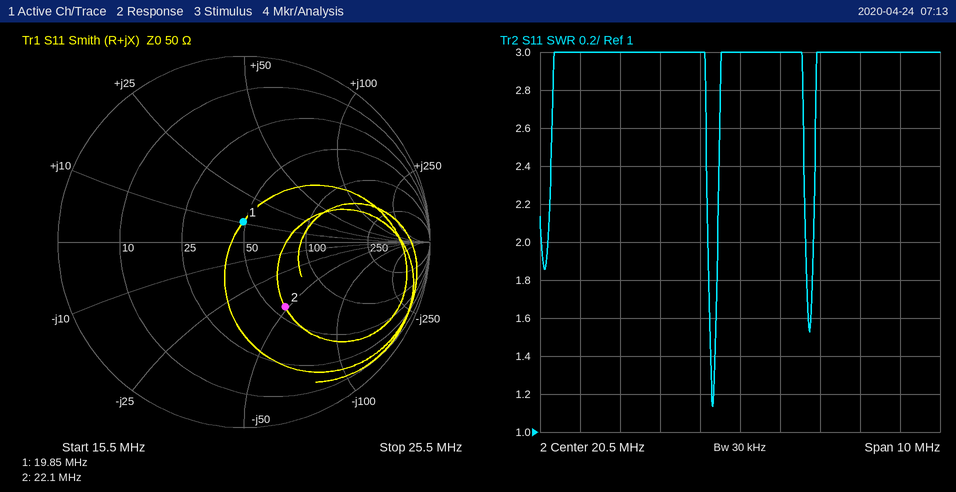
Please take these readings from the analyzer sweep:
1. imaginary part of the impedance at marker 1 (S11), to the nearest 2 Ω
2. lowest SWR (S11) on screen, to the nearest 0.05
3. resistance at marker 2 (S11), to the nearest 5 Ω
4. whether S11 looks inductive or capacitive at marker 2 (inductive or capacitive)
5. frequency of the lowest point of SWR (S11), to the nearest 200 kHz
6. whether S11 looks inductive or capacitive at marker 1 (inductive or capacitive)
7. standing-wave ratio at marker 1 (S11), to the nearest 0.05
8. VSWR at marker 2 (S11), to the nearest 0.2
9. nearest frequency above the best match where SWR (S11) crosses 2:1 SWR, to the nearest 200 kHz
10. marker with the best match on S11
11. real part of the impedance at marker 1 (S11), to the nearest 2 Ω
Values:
+10 Ω
1.15
55 Ω
capacitive
19.8 MHz
inductive
1.25
2.4
20.0 MHz
marker 1
48 Ω
